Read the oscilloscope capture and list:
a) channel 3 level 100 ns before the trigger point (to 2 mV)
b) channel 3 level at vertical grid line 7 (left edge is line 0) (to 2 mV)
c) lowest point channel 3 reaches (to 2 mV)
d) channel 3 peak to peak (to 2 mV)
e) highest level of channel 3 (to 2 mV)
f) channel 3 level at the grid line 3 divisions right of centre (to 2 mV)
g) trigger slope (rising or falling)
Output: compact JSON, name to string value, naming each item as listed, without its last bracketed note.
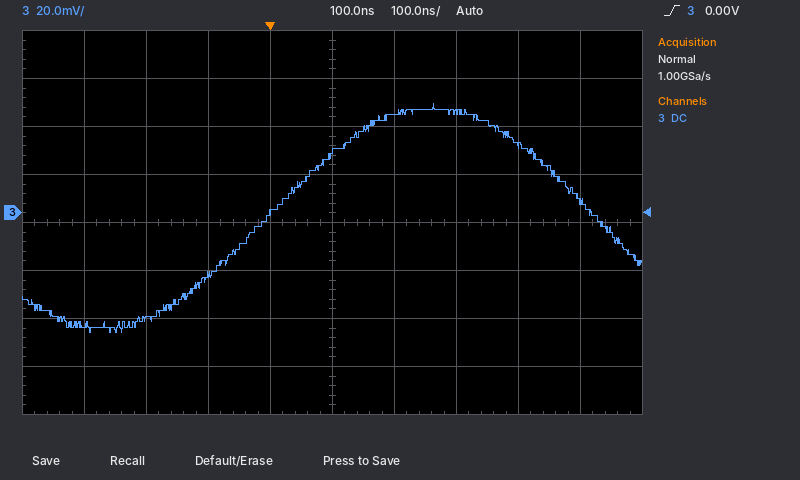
{"channel 3 level 100 ns before the trigger point": "-26 mV", "channel 3 level at vertical grid line 7 (left edge is line 0)": "42 mV", "lowest point channel 3 reaches": "-50 mV", "channel 3 peak to peak": "96 mV", "highest level of channel 3": "46 mV", "channel 3 level at the grid line 3 divisions right of centre": "28 mV", "trigger slope": "rising"}
